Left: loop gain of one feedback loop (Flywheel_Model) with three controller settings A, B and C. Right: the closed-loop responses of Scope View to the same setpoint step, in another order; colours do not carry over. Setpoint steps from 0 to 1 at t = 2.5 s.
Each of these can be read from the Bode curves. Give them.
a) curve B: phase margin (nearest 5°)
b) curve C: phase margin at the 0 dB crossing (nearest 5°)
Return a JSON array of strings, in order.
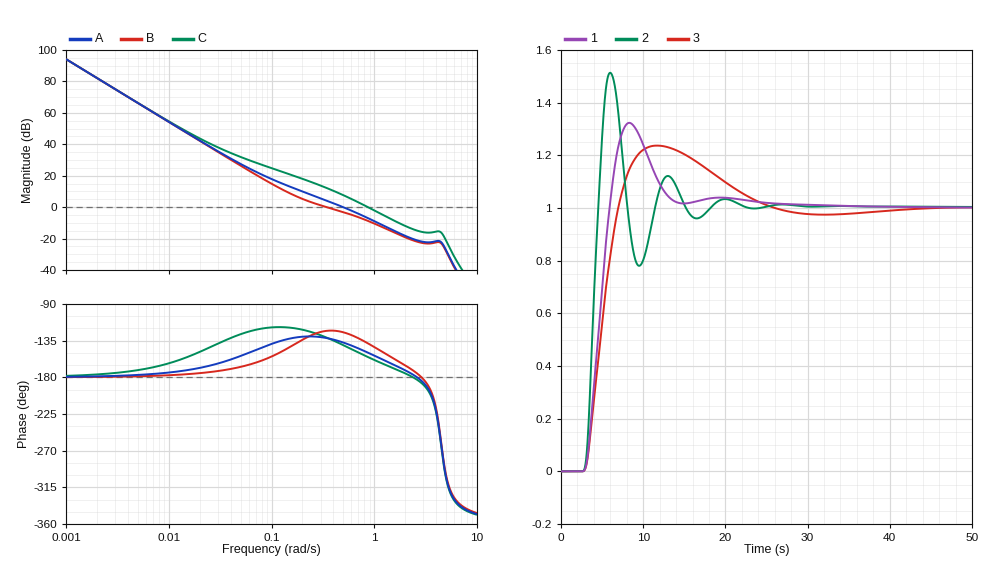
["55°", "25°"]
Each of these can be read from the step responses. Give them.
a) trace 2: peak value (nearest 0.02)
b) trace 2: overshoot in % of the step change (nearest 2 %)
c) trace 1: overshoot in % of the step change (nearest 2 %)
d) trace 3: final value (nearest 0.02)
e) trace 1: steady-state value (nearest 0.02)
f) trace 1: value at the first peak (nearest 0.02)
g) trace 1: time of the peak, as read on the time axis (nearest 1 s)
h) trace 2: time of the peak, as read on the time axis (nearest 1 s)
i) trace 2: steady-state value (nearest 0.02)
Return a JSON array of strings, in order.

["1.52", "52 %", "32 %", "1.00", "1.00", "1.32", "8 s", "6 s", "1.00"]
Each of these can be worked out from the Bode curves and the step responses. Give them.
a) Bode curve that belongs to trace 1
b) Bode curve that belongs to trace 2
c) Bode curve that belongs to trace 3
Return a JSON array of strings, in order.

["A", "C", "B"]
